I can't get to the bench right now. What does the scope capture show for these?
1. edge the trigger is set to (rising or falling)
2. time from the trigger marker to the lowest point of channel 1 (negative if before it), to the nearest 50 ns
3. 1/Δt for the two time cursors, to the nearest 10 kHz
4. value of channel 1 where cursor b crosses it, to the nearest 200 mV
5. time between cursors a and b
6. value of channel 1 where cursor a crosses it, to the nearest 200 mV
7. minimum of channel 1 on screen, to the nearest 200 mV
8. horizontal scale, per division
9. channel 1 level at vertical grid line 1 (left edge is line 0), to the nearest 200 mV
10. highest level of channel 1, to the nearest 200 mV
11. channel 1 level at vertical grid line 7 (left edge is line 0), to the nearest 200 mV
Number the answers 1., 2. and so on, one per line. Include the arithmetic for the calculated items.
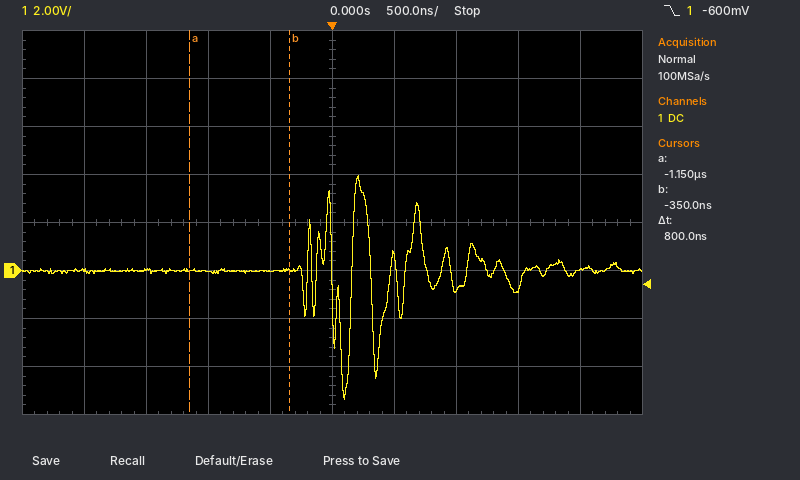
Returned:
1. falling
2. +100 ns
3. 1 / 800 ns ≈ 1.25 MHz
4. 0.0 V
5. 800 ns
6. 0.0 V
7. -5.4 V
8. 500 ns
9. 0.0 V
10. 4.0 V
11. -800 mV
